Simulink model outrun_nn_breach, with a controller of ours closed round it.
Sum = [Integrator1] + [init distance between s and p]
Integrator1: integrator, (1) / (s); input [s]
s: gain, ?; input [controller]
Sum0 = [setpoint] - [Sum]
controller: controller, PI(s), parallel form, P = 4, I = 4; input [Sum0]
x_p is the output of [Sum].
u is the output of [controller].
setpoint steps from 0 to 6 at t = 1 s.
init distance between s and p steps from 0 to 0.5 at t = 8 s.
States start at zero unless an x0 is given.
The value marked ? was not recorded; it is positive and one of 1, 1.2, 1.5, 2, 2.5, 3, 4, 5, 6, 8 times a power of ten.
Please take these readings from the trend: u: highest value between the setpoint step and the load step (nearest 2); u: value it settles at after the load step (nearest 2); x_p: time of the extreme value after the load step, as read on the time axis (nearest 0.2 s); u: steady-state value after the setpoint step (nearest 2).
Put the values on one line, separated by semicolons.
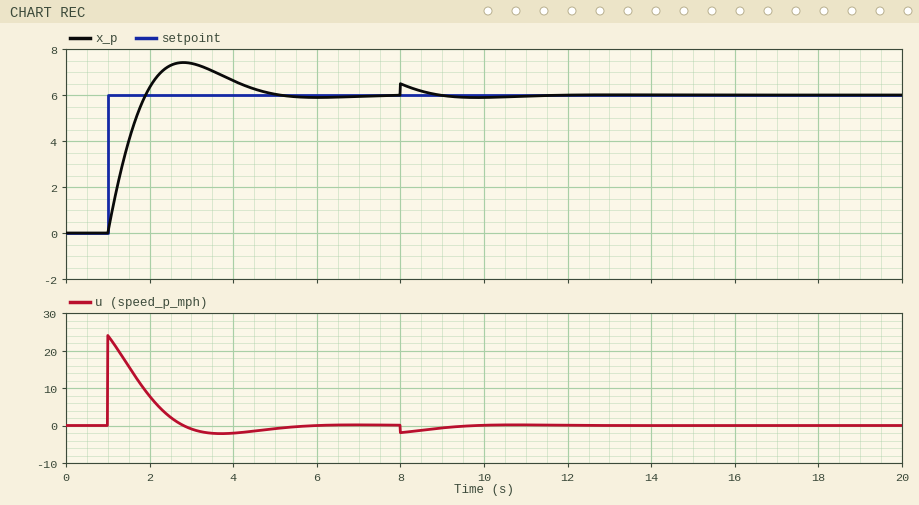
24; 0; 8.0 s; 0
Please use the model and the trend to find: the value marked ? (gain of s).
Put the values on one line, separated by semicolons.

0.4
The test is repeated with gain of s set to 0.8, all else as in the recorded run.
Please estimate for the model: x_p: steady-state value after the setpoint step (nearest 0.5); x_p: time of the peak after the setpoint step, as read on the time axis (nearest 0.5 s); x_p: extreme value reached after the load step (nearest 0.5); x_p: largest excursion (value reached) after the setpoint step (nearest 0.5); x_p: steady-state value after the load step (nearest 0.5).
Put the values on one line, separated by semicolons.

6.0; 2.0 s; 6.5; 7.0; 6.0
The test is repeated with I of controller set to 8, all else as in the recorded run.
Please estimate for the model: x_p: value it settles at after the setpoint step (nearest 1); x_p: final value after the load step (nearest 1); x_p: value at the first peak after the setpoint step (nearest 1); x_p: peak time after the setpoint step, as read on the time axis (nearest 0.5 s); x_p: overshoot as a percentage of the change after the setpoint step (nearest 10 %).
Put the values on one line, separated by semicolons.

6; 6; 8; 2.5 s; 30 %
